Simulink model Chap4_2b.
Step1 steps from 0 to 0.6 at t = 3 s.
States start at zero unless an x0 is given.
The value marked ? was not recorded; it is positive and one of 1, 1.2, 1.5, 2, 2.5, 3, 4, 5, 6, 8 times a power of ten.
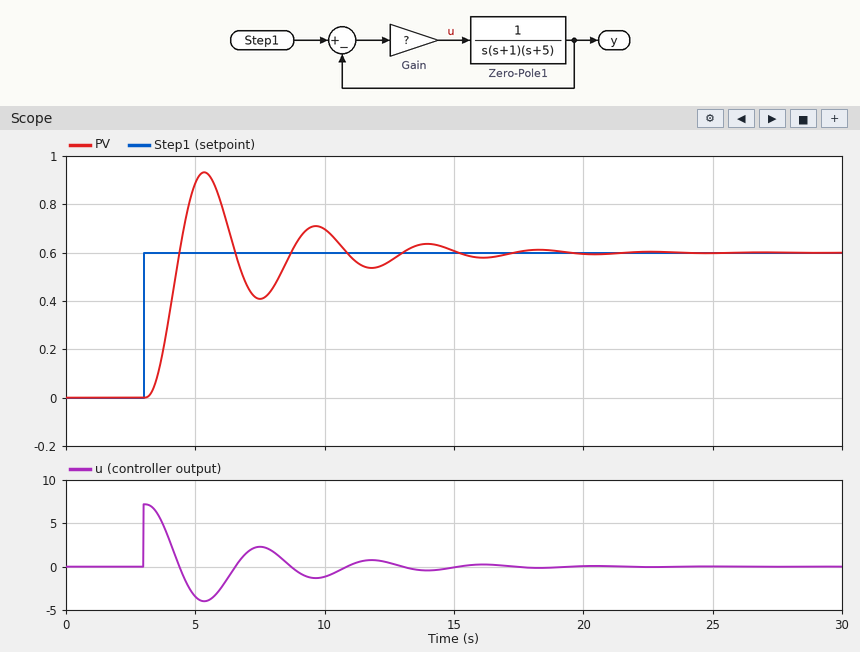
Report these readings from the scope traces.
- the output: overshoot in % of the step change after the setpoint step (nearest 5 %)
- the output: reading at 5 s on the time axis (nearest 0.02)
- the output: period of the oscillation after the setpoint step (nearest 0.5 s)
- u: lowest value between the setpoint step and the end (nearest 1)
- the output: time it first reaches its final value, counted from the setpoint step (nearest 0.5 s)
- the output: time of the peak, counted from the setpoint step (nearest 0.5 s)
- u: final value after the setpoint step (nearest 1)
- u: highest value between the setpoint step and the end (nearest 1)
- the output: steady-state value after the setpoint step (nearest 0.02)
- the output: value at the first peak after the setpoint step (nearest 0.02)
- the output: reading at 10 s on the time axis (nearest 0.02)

55 %
0.88
4.5 s
-4
1.5 s
2.5 s
0
7
0.60
0.94
0.70
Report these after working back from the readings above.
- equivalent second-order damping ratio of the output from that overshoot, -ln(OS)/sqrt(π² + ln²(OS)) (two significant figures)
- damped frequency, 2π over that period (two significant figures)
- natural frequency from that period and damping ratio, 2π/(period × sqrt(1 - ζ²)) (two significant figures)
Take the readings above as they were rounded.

0.19
1.4 rad/s
1.4 rad/s
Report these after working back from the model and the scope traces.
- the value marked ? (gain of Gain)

12
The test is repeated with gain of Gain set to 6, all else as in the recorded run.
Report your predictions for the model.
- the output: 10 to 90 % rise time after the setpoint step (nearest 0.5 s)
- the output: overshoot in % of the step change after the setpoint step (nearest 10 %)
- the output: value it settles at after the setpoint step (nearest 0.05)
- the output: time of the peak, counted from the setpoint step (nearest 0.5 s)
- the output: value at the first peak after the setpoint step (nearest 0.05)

1.5 s
30 %
0.60
3.5 s
0.80
